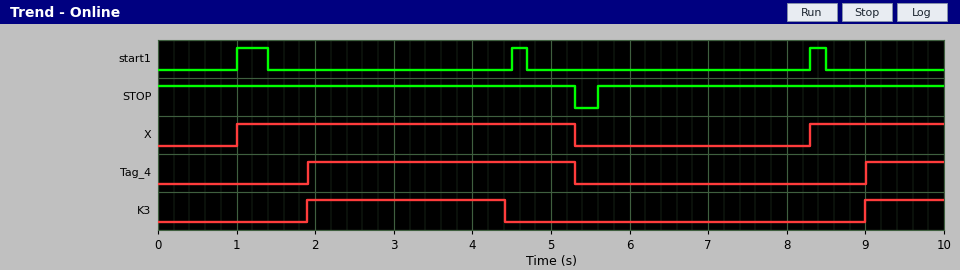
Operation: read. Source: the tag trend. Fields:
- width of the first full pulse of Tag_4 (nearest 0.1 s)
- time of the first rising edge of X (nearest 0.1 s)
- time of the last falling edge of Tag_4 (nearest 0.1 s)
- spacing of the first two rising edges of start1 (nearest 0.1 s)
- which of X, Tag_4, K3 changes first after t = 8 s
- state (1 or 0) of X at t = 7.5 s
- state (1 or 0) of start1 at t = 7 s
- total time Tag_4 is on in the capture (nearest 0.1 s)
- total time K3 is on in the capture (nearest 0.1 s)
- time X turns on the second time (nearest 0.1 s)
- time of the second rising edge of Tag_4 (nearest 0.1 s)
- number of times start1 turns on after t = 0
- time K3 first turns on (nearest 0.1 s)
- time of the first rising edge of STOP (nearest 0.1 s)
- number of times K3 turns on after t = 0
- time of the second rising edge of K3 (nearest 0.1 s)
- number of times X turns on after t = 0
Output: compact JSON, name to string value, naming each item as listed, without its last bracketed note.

{"width of the first full pulse of Tag_4": "3.4 s", "time of the first rising edge of X": "1.0 s", "time of the last falling edge of Tag_4": "5.3 s", "spacing of the first two rising edges of start1": "3.5 s", "which of X, Tag_4, K3 changes first after t = 8 s": "X", "state (1 or 0) of X at t = 7.5 s": "0", "state (1 or 0) of start1 at t = 7 s": "0", "total time Tag_4 is on in the capture": "4.4 s", "total time K3 is on in the capture": "3.5 s", "time X turns on the second time": "8.3 s", "time of the second rising edge of Tag_4": "9.0 s", "number of times start1 turns on after t = 0": "3", "time K3 first turns on": "1.9 s", "time of the first rising edge of STOP": "5.6 s", "number of times K3 turns on after t = 0": "2", "time of the second rising edge of K3": "9.0 s", "number of times X turns on after t = 0": "2"}
